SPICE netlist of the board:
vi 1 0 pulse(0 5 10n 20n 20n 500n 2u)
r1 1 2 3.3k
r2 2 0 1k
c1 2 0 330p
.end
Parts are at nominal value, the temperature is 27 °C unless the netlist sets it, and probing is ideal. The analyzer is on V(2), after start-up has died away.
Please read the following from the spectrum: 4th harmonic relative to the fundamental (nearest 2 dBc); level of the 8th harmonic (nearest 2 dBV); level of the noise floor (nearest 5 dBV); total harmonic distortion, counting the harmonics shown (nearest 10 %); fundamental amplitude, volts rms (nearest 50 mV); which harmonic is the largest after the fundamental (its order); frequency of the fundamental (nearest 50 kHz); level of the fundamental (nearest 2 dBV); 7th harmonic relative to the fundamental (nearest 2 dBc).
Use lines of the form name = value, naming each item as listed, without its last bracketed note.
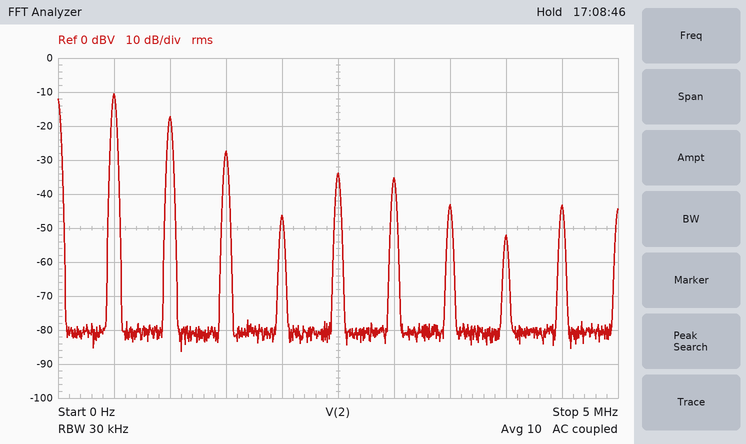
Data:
4th harmonic relative to the fundamental = -36 dBc
level of the 8th harmonic = -52 dBV
level of the noise floor = -80 dBV
total harmonic distortion, counting the harmonics shown = 50 %
fundamental amplitude, volts rms = 300 mV
which harmonic is the largest after the fundamental = 2
frequency of the fundamental = 500 kHz
level of the fundamental = -10 dBV
7th harmonic relative to the fundamental = -32 dBc
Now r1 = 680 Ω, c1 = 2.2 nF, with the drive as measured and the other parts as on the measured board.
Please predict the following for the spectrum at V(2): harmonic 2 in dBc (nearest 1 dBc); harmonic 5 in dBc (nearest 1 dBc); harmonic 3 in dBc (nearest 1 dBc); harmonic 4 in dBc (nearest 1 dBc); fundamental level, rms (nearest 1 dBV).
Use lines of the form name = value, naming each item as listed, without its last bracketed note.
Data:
harmonic 2 in dBc = -9 dBc
harmonic 5 in dBc = -27 dBc
harmonic 3 in dBc = -20 dBc
harmonic 4 in dBc = -39 dBc
fundamental level, rms = -10 dBV
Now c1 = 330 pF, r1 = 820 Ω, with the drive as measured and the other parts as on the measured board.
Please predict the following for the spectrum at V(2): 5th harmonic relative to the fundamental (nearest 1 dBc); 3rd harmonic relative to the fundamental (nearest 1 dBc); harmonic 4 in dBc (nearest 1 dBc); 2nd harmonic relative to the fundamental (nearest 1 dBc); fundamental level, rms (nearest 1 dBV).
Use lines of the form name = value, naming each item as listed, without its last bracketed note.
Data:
5th harmonic relative to the fundamental = -20 dBc
3rd harmonic relative to the fundamental = -15 dBc
harmonic 4 in dBc = -33 dBc
2nd harmonic relative to the fundamental = -5 dBc
fundamental level, rms = -2 dBV
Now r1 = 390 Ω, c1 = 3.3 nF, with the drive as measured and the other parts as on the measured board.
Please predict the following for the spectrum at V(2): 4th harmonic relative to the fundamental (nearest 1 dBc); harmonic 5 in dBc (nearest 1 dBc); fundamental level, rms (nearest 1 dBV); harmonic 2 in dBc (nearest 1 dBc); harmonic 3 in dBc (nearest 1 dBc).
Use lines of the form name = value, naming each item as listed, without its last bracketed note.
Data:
4th harmonic relative to the fundamental = -39 dBc
harmonic 5 in dBc = -27 dBc
fundamental level, rms = -8 dBV
harmonic 2 in dBc = -9 dBc
harmonic 3 in dBc = -20 dBc
